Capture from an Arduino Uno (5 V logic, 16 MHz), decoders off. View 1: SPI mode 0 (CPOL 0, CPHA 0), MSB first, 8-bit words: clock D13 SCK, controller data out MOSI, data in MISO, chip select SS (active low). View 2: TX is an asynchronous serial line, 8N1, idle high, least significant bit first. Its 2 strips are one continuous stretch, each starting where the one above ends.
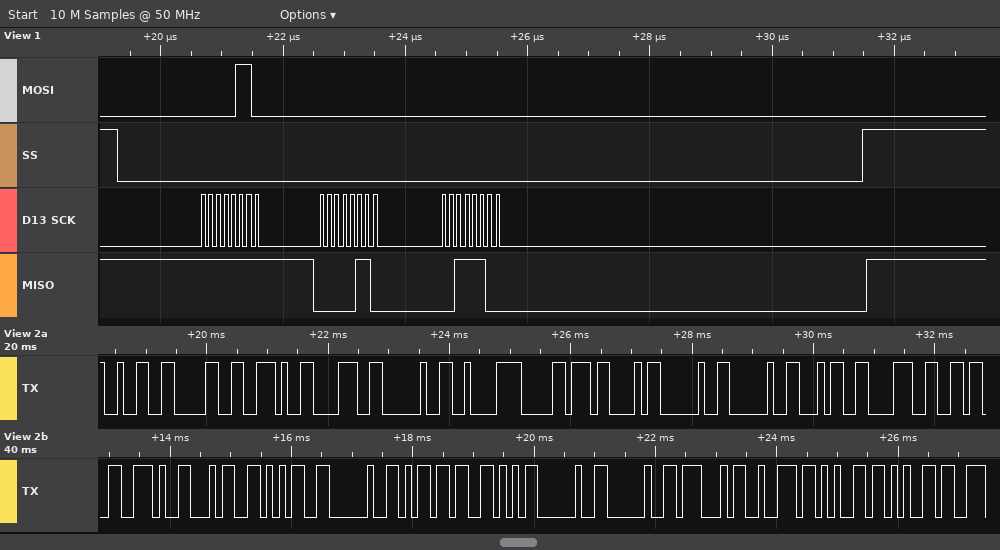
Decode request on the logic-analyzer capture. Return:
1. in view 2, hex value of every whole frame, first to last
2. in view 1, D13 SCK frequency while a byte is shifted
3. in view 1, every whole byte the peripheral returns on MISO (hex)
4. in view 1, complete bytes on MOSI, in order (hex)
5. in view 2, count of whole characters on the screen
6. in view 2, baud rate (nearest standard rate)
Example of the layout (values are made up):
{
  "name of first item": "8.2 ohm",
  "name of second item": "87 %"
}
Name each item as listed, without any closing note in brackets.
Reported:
{
  "in view 2, hex value of every whole frame, first to last": "32 30 2E 38 20 C2 B0 43 20 20 34 38 36 2E 34 35 20 6D 56 20 20 47 72 65 65",
  "in view 1, D13 SCK frequency while a byte is shifted": "8 MHz",
  "in view 1, every whole byte the peripheral returns on MISO": "0xFF 0x06 0x3C",
  "in view 1, complete bytes on MOSI, in order": "0x06 0x00 0x00",
  "in view 2, count of whole characters on the screen": "25",
  "in view 2, baud rate": "9600 baud"
}
